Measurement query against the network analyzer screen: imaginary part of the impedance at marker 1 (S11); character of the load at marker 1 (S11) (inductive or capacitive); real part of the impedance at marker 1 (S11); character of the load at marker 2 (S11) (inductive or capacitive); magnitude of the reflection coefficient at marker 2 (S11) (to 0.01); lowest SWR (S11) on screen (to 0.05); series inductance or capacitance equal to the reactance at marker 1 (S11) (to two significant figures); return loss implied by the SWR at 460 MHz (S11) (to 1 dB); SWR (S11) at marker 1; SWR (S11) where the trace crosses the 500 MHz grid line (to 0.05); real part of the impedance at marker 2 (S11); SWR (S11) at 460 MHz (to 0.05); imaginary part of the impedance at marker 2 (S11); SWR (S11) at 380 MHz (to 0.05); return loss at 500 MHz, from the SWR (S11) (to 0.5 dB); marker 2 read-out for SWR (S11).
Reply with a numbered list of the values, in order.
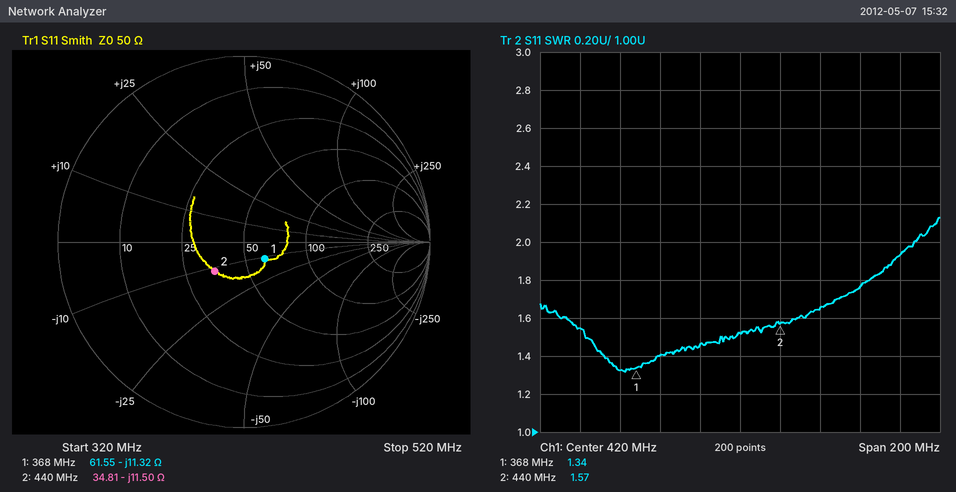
1. -11.32 Ω
2. capacitive
3. 61.55 Ω
4. capacitive
5. 0.22
6. 1.30
7. 38 pF
8. 12 dB
9. 1.34
10. 1.95
11. 34.81 Ω
12. 1.65
13. -11.50 Ω
14. 1.40
15. 10.0 dB
16. 1.57
